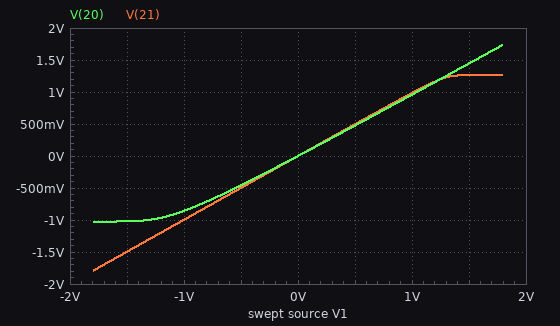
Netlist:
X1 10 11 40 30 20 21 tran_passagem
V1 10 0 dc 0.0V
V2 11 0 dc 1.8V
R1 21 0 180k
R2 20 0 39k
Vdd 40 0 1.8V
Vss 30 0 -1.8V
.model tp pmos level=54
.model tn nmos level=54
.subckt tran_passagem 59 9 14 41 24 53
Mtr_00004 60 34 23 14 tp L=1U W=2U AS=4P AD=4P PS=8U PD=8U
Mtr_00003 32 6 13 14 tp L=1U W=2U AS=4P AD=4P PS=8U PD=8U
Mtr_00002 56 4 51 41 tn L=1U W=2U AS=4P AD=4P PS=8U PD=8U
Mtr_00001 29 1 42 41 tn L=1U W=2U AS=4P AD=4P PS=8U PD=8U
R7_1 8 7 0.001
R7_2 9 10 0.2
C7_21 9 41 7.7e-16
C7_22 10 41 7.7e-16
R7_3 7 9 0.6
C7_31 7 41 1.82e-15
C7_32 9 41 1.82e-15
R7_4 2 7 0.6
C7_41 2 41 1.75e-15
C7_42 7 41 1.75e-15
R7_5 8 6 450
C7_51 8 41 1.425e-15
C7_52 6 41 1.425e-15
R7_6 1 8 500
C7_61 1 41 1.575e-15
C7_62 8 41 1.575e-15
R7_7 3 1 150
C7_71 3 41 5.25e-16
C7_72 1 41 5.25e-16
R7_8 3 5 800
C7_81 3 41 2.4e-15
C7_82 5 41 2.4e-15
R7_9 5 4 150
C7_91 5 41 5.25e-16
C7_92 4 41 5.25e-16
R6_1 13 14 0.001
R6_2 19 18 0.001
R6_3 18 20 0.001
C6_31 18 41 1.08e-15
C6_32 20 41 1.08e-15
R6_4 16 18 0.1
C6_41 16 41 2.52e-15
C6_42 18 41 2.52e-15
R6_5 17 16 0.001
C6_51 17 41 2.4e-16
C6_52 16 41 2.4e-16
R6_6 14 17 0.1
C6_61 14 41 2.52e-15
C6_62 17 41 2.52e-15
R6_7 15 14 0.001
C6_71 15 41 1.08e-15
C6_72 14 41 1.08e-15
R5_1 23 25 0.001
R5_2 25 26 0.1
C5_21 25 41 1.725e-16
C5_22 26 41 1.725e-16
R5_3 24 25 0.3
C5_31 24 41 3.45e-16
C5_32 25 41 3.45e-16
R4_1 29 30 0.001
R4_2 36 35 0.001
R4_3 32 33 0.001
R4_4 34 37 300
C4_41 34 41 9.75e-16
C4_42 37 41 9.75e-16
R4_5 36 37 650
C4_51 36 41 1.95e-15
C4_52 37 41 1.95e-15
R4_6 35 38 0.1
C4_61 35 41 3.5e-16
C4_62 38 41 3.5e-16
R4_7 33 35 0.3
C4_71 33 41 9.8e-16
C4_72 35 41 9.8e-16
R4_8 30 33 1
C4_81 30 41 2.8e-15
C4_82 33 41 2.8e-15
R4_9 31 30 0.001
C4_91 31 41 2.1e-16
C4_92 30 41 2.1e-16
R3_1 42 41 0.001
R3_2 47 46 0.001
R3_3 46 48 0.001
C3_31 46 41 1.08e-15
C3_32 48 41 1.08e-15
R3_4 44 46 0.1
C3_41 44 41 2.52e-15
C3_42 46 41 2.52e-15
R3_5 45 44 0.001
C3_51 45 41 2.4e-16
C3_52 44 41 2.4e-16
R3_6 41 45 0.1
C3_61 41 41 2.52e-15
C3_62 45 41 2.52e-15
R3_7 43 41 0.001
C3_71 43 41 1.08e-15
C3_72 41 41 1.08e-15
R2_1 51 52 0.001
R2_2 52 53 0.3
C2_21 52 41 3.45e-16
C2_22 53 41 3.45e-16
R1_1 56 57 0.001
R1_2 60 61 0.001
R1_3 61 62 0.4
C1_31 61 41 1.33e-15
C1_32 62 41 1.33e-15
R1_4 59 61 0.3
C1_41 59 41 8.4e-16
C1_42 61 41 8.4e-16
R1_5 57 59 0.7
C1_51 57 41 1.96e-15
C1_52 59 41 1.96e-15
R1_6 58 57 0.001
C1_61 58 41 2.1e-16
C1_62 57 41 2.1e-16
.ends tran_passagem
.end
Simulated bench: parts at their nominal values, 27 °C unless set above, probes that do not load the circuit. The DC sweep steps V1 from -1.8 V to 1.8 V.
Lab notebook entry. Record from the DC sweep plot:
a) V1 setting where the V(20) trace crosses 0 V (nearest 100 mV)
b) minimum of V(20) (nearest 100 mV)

0 V
-1.0 V
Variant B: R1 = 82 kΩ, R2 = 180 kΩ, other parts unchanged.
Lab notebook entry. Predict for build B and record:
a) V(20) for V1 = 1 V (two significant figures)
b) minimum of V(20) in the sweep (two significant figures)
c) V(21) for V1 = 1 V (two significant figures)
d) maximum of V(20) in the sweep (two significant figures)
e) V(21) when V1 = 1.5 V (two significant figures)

990 mV
-1.2 V
970 mV
1.8 V
1.2 V
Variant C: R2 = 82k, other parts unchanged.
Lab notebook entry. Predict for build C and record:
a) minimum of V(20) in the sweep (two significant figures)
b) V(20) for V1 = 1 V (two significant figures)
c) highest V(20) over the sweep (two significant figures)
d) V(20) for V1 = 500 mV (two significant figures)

-1.1 V
980 mV
1.8 V
490 mV
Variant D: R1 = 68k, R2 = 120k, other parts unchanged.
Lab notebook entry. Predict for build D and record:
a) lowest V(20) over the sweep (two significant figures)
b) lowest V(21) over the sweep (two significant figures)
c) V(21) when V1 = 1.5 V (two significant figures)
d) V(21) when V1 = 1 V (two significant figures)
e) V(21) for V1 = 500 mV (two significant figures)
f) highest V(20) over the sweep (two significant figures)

-1.2 V
-1.8 V
1.2 V
960 mV
490 mV
1.8 V
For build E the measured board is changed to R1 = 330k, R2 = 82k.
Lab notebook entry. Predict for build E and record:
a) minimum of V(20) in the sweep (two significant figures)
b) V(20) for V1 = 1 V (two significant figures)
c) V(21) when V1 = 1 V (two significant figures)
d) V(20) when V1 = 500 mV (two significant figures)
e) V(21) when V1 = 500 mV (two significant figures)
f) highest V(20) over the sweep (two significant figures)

-1.1 V
980 mV
990 mV
490 mV
500 mV
1.8 V
